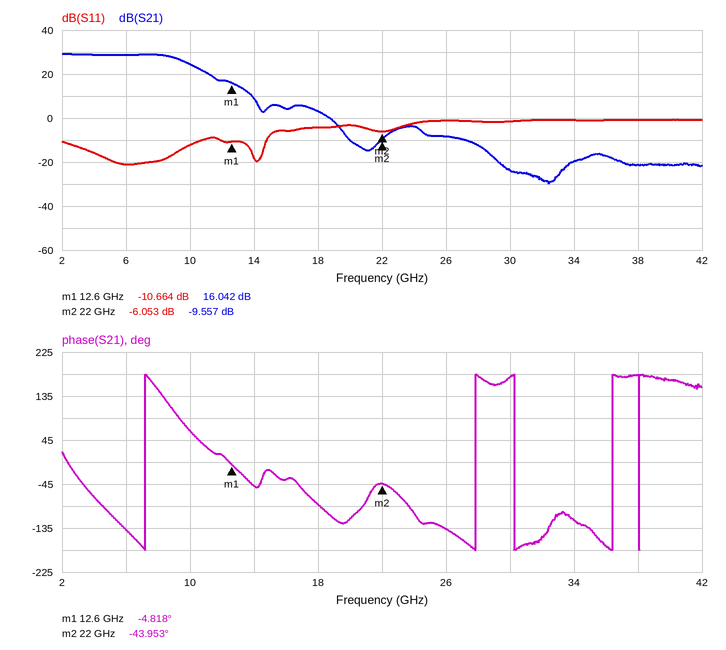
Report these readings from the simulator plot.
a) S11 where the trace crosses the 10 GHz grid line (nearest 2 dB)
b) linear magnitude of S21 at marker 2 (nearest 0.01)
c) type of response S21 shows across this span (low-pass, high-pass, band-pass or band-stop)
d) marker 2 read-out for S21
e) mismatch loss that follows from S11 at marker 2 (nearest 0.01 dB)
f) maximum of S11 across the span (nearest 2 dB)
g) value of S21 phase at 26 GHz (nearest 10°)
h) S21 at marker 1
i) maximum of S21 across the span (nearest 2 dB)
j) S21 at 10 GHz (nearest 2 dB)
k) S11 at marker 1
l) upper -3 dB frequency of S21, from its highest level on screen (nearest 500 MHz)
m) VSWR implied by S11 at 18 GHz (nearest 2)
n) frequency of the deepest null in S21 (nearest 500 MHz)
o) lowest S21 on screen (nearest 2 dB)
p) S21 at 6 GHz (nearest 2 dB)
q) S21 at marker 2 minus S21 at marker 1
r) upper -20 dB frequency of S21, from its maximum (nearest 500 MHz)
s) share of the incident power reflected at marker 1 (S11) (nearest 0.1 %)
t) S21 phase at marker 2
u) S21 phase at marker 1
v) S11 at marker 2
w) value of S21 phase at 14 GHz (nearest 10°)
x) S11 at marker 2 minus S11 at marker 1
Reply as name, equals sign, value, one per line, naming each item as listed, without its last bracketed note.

S11 where the trace crosses the 10 GHz grid line = -12 dB
linear magnitude of S21 at marker 2 = 0.33
type of response S21 shows across this span = low-pass
marker 2 read-out for S21 = -9.557 dB
mismatch loss that follows from S11 at marker 2 = 1.24 dB
maximum of S11 across the span = 0 dB
value of S21 phase at 26 GHz = -140°
S21 at marker 1 = 16.042 dB
maximum of S21 across the span = 30 dB
S21 at 10 GHz = 24 dB
S11 at marker 1 = -10.664 dB
upper -3 dB frequency of S21, from its highest level on screen = 9.5 GHz
VSWR implied by S11 at 18 GHz = 4
frequency of the deepest null in S21 = 32.5 GHz
lowest S21 on screen = -30 dB
S21 at 6 GHz = 28 dB
S21 at marker 2 minus S21 at marker 1 = -25.599 dB
upper -20 dB frequency of S21, from its maximum = 14.0 GHz
share of the incident power reflected at marker 1 (S11) = 8.6 %
S21 phase at marker 2 = -43.953°
S21 phase at marker 1 = -4.818°
S11 at marker 2 = -6.053 dB
value of S21 phase at 14 GHz = -50°
S11 at marker 2 minus S11 at marker 1 = 4.611 dB
